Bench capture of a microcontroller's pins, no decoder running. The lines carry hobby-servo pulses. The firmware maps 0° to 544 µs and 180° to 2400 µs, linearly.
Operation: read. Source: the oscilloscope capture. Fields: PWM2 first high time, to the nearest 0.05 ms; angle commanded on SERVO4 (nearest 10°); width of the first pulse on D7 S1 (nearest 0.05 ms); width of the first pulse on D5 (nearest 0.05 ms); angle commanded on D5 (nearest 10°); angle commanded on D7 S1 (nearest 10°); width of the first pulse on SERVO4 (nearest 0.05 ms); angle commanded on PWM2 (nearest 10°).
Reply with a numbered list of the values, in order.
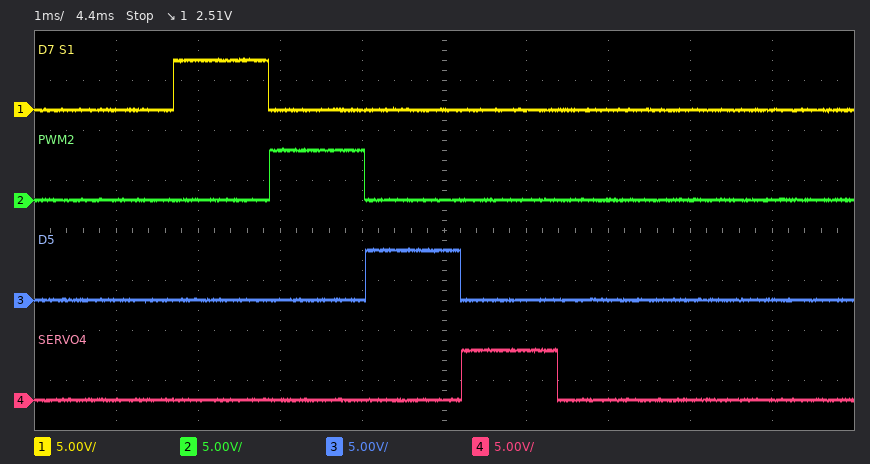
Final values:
1. 1.15 ms
2. 60°
3. 1.15 ms
4. 1.15 ms
5. 60°
6. 60°
7. 1.15 ms
8. 60°
